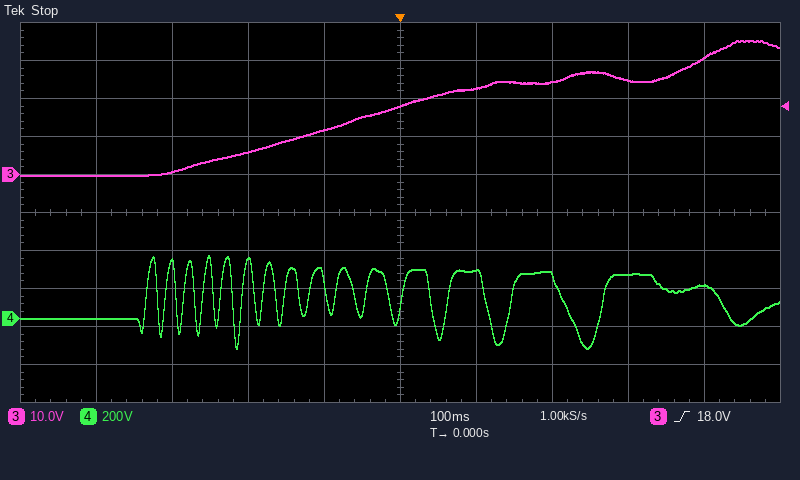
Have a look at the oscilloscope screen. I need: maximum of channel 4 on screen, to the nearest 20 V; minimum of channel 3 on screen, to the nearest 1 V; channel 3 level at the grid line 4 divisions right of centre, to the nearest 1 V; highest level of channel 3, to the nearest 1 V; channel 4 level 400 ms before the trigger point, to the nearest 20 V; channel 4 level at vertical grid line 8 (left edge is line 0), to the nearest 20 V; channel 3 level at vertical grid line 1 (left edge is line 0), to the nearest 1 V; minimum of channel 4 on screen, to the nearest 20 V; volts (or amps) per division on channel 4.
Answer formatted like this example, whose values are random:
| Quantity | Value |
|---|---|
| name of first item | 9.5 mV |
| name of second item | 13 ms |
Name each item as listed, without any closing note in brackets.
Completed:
| Quantity | Value |
|---|---|
| maximum of channel 4 on screen, to the nearest 20 V | 340 V |
| minimum of channel 3 on screen, to the nearest 1 V | 0 V |
| channel 3 level at the grid line 4 divisions right of centre, to the nearest 1 V | 31 V |
| highest level of channel 3, to the nearest 1 V | 35 V |
| channel 4 level 400 ms before the trigger point, to the nearest 20 V | 0 V |
| channel 4 level at vertical grid line 8 (left edge is line 0), to the nearest 20 V | 240 V |
| channel 3 level at vertical grid line 1 (left edge is line 0), to the nearest 1 V | 0 V |
| minimum of channel 4 on screen, to the nearest 20 V | -160 V |
| volts (or amps) per division on channel 4 | 200 V |
